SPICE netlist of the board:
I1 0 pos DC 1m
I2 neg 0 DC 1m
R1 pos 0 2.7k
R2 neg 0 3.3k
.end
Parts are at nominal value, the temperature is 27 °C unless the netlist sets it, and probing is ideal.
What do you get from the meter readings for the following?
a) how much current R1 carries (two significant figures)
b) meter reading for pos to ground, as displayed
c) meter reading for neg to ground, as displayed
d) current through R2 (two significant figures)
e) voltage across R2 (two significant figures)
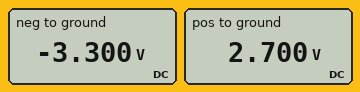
1.0 mA
2.700 V
-3.300 V
1.0 mA
3.3 V
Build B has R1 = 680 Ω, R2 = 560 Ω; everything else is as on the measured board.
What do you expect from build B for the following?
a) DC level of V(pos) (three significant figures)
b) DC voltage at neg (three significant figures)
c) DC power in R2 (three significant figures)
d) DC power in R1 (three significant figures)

680 mV
-560 mV
560 µW
680 µW
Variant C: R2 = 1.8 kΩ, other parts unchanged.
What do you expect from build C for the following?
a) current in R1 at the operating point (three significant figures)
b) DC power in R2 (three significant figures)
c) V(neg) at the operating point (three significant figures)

1.00 mA
1.80 mW
-1.80 V
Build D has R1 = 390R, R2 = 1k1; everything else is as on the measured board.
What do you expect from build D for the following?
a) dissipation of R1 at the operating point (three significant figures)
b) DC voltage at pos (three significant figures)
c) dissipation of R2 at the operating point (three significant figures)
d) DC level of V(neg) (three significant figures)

390 µW
390 mV
1.10 mW
-1.10 V
